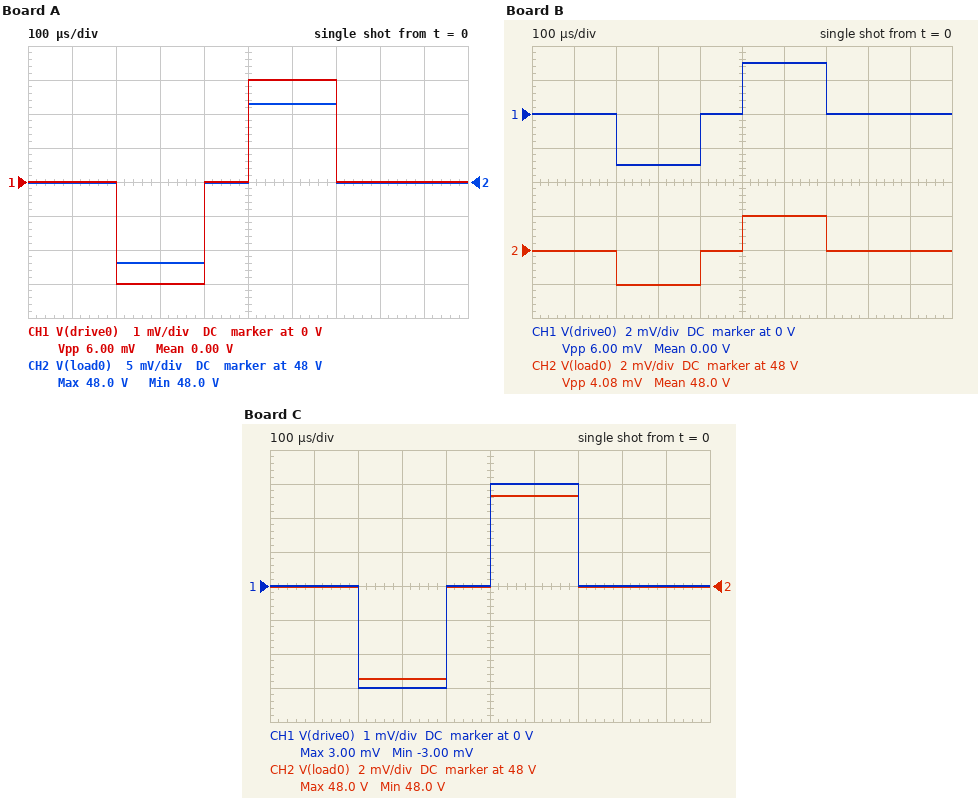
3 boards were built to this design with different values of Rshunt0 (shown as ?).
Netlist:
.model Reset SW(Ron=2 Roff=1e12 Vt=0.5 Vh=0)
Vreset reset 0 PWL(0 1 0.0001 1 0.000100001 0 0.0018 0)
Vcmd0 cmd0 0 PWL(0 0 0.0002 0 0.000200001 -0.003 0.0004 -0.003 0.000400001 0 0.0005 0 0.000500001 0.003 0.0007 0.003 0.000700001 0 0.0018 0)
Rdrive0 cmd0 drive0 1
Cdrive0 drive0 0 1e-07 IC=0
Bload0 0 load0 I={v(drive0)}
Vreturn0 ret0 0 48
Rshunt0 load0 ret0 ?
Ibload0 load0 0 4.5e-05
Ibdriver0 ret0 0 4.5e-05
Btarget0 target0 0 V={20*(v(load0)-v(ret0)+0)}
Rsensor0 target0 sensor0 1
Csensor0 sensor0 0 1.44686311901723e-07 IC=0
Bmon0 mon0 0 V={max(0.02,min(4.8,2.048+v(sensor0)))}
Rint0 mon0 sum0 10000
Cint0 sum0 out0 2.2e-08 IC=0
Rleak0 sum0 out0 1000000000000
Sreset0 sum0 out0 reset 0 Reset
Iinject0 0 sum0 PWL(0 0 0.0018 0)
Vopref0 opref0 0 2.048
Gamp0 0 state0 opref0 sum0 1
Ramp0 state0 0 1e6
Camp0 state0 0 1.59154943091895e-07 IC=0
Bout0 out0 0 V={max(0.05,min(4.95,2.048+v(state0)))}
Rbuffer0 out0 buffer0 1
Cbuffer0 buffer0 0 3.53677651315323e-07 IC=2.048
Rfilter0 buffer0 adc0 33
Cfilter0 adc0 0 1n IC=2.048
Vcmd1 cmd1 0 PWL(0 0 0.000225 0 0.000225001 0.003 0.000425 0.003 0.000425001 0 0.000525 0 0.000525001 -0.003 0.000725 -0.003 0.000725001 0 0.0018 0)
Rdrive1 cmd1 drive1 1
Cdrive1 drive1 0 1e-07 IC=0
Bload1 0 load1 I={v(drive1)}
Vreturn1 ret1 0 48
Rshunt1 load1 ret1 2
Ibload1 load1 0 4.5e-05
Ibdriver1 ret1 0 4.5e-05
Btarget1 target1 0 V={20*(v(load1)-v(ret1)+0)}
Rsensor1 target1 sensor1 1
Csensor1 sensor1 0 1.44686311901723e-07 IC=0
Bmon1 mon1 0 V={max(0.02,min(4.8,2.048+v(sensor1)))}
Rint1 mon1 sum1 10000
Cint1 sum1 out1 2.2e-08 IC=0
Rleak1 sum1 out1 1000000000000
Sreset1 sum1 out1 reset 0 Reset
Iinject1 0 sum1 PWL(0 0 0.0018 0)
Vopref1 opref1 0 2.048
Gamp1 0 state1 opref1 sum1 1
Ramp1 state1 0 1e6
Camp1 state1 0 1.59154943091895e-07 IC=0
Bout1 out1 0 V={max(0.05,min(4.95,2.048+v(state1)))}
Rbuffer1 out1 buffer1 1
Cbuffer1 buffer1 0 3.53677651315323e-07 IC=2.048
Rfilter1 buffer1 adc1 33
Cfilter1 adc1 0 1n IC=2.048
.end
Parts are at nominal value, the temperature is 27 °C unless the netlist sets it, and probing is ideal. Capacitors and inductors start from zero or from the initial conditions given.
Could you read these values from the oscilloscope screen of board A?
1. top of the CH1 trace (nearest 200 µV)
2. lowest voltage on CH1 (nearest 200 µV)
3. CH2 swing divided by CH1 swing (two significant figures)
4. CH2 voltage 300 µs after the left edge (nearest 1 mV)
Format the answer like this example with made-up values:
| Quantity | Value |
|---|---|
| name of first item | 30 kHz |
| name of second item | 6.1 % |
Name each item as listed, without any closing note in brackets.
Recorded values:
| Quantity | Value |
|---|---|
| top of the CH1 trace | 3.0 mV |
| lowest voltage on CH1 | -3.0 mV |
| CH2 swing divided by CH1 swing | 3.9 |
| CH2 voltage 300 µs after the left edge | 47.988 V |
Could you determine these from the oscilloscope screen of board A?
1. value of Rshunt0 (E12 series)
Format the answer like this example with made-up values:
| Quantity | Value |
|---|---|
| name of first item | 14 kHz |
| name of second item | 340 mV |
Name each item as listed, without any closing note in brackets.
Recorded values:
| Quantity | Value |
|---|---|
| value of Rshunt0 | 3.9 Ω |
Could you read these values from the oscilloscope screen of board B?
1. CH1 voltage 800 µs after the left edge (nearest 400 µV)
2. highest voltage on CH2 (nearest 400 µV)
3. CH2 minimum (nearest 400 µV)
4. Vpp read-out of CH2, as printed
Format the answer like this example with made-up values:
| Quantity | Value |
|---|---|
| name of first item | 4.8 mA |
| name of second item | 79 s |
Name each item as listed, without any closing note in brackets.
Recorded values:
| Quantity | Value |
|---|---|
| CH1 voltage 800 µs after the left edge | 0 V |
| highest voltage on CH2 | 48.0020 V |
| CH2 minimum | 47.9980 V |
| Vpp read-out of CH2, as printed | 4.08 mV |
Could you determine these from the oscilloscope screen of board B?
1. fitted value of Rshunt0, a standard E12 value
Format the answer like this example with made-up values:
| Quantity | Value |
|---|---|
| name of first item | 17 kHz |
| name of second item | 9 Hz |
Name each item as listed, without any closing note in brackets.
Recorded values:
| Quantity | Value |
|---|---|
| fitted value of Rshunt0, a standard E12 value | 0.68 Ω |
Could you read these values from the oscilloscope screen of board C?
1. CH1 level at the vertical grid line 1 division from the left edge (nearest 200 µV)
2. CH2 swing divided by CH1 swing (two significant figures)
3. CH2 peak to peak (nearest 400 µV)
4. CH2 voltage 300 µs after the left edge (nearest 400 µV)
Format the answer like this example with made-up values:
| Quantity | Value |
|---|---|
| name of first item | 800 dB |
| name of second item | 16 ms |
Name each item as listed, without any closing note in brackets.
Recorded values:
| Quantity | Value |
|---|---|
| CH1 level at the vertical grid line 1 division from the left edge | 0 V |
| CH2 swing divided by CH1 swing | 1.8 |
| CH2 peak to peak | 10.8 mV |
| CH2 voltage 300 µs after the left edge | 47.9944 V |
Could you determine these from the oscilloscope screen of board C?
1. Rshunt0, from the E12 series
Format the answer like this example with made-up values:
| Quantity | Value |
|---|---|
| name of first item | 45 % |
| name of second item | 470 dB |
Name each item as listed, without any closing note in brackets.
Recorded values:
| Quantity | Value |
|---|---|
| Rshunt0, from the E12 series | 1.8 Ω |
